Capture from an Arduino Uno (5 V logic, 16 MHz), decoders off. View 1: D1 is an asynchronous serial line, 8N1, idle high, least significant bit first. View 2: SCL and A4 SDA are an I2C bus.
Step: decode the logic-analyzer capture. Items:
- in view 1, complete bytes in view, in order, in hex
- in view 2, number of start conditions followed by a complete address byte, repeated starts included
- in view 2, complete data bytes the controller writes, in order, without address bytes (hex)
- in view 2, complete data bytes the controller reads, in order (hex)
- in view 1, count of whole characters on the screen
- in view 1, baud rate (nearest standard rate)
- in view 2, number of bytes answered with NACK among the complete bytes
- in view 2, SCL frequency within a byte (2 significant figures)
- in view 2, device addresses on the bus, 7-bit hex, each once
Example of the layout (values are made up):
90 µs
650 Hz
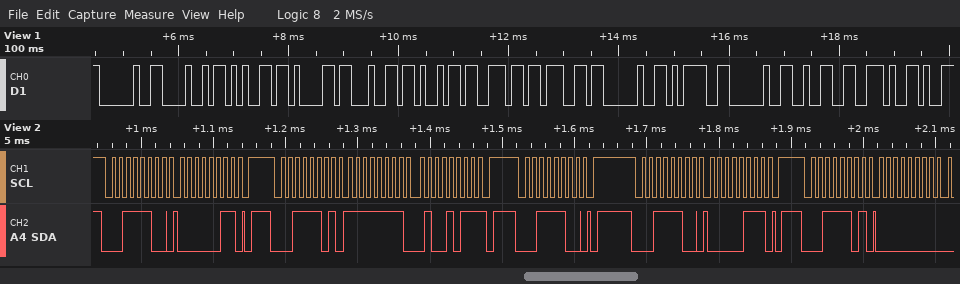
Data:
20 48 65 61 64 69 6E 67 20 3D 20 32 2E
5
03 07
FF 4B 00
13
9600 baud
1
100 kHz
0x1E
